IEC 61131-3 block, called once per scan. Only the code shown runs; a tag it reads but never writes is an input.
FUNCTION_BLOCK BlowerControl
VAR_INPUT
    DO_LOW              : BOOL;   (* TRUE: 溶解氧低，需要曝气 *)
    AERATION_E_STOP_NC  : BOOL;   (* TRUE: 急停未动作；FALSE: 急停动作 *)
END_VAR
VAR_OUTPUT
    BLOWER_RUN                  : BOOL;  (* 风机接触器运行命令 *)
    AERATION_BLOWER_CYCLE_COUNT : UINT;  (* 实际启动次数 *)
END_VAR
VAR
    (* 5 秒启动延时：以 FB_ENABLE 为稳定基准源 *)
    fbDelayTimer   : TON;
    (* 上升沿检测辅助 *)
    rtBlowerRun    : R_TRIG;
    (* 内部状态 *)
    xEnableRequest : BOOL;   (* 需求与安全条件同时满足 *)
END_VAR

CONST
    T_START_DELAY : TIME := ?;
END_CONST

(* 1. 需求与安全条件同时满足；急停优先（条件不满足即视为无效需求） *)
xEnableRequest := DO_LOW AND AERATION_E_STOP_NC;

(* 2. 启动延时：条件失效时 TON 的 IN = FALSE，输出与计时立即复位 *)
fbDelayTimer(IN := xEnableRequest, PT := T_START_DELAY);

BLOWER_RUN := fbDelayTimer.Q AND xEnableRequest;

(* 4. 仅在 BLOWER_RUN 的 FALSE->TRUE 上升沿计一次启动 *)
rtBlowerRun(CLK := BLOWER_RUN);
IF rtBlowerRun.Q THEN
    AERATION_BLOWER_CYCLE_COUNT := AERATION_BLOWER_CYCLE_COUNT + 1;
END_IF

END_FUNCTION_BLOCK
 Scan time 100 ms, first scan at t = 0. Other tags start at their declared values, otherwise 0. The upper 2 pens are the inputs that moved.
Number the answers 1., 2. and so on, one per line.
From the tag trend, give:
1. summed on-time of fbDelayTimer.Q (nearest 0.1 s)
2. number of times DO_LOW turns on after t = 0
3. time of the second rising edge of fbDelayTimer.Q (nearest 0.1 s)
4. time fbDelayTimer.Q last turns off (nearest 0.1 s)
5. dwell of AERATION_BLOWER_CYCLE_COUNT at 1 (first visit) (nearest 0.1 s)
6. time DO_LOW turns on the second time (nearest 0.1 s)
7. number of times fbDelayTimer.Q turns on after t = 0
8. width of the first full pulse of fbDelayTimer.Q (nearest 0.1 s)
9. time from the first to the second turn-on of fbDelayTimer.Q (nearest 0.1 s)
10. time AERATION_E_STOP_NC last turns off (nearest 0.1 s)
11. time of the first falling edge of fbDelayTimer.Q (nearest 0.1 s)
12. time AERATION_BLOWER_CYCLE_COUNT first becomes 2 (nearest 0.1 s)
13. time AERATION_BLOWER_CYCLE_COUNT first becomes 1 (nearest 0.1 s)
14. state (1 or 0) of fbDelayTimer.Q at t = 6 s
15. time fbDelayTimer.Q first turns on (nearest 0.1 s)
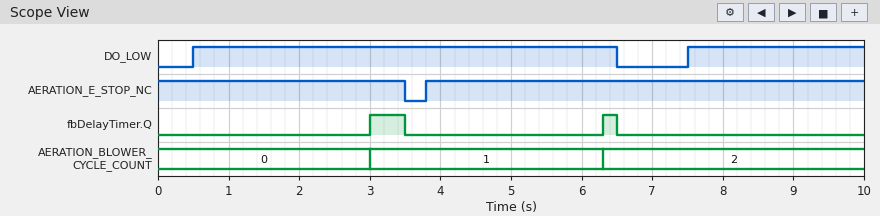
1. 0.7 s
2. 2
3. 6.3 s
4. 6.5 s
5. 3.3 s
6. 7.5 s
7. 2
8. 0.5 s
9. 3.3 s
10. 3.5 s
11. 3.5 s
12. 6.3 s
13. 3.0 s
14. 0
15. 3.0 s
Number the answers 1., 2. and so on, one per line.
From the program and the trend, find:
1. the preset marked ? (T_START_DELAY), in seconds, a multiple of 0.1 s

1. 2.5 s
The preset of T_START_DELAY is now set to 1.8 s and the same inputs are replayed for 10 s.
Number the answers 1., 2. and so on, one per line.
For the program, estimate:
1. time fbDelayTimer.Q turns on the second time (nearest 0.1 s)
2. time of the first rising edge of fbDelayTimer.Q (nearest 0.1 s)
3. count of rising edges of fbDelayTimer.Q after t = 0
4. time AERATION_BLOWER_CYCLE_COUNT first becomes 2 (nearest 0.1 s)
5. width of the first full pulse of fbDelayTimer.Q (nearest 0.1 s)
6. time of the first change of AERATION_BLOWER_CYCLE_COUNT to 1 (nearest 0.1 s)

1. 5.6 s
2. 2.3 s
3. 3
4. 5.6 s
5. 1.2 s
6. 2.3 s
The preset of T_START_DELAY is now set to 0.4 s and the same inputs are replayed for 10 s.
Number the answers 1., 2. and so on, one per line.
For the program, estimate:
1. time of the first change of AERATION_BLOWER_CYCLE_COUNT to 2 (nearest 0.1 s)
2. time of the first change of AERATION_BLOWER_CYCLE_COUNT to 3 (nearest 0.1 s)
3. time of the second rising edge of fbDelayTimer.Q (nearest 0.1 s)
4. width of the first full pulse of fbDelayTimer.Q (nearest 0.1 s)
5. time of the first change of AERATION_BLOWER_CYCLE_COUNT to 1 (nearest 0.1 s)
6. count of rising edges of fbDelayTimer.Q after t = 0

1. 4.2 s
2. 7.9 s
3. 4.2 s
4. 2.6 s
5. 0.9 s
6. 3
